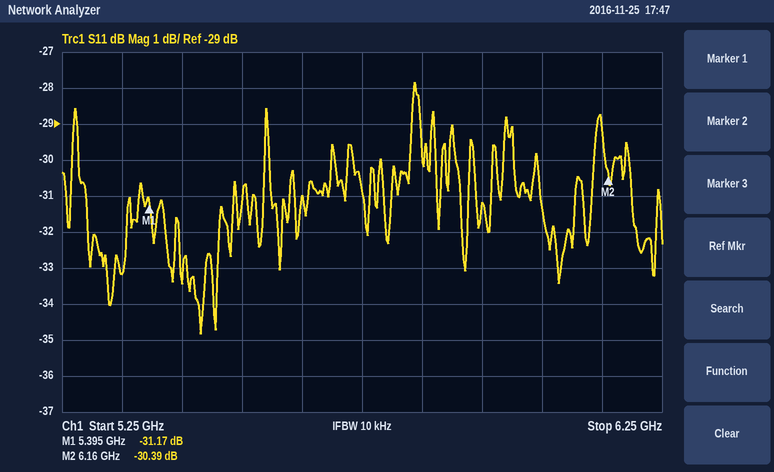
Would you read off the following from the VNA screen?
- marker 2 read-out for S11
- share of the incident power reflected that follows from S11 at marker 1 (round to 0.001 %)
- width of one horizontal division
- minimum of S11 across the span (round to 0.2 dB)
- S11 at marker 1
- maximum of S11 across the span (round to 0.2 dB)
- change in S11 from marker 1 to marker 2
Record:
-30.39 dB
0.076 %
100 MHz
-34.8 dB
-31.17 dB
-27.8 dB
0.78 dB
